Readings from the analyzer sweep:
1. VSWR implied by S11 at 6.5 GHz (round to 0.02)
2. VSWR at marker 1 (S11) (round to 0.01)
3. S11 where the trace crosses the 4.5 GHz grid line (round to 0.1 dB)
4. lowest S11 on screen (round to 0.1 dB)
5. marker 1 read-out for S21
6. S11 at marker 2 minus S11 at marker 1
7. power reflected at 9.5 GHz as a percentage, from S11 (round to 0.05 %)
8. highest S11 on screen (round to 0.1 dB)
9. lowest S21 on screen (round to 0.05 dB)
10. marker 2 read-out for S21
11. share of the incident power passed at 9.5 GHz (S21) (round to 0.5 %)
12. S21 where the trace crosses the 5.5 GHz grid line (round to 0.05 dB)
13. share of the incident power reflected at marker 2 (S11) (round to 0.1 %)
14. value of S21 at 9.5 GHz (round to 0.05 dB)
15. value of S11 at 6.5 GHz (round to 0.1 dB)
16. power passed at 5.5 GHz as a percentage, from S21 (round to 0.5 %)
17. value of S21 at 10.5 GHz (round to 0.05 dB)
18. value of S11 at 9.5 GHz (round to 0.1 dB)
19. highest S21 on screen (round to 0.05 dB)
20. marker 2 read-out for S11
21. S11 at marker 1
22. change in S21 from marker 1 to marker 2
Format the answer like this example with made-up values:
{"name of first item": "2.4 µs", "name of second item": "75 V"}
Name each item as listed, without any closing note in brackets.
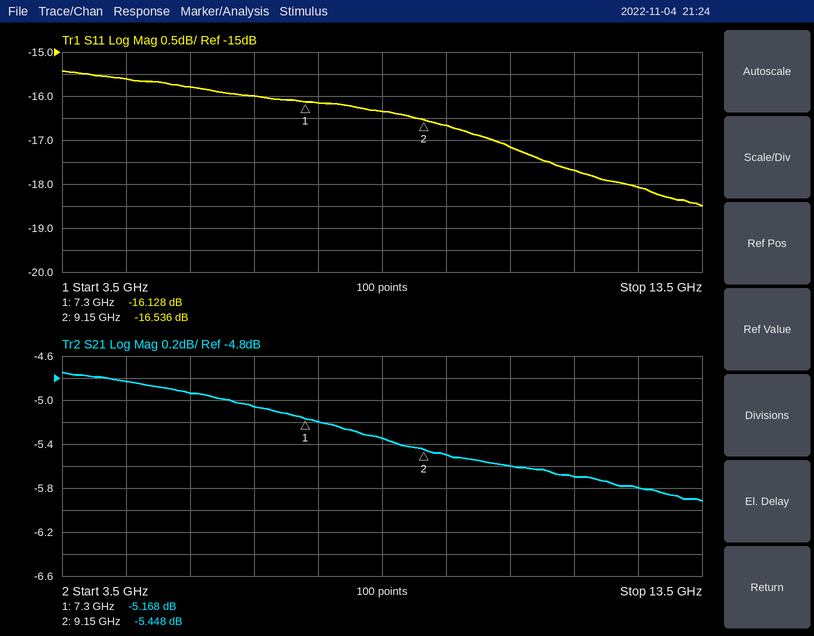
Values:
{"VSWR implied by S11 at 6.5 GHz": "1.38", "VSWR at marker 1 (S11)": "1.37", "S11 where the trace crosses the 4.5 GHz grid line": "-15.6 dB", "lowest S11 on screen": "-18.5 dB", "marker 1 read-out for S21": "-5.168 dB", "S11 at marker 2 minus S11 at marker 1": "-0.408 dB", "power reflected at 9.5 GHz as a percentage, from S11": "2.15 %", "highest S11 on screen": "-15.4 dB", "lowest S21 on screen": "-5.90 dB", "marker 2 read-out for S21": "-5.448 dB", "share of the incident power passed at 9.5 GHz (S21)": "28.0 %", "S21 where the trace crosses the 5.5 GHz grid line": "-4.95 dB", "share of the incident power reflected at marker 2 (S11)": "2.2 %", "value of S21 at 9.5 GHz": "-5.50 dB", "value of S11 at 6.5 GHz": "-16.0 dB", "power passed at 5.5 GHz as a percentage, from S21": "32.0 %", "value of S21 at 10.5 GHz": "-5.60 dB", "value of S11 at 9.5 GHz": "-16.7 dB", "highest S21 on screen": "-4.75 dB", "marker 2 read-out for S11": "-16.536 dB", "S11 at marker 1": "-16.128 dB", "change in S21 from marker 1 to marker 2": "-0.280 dB"}
